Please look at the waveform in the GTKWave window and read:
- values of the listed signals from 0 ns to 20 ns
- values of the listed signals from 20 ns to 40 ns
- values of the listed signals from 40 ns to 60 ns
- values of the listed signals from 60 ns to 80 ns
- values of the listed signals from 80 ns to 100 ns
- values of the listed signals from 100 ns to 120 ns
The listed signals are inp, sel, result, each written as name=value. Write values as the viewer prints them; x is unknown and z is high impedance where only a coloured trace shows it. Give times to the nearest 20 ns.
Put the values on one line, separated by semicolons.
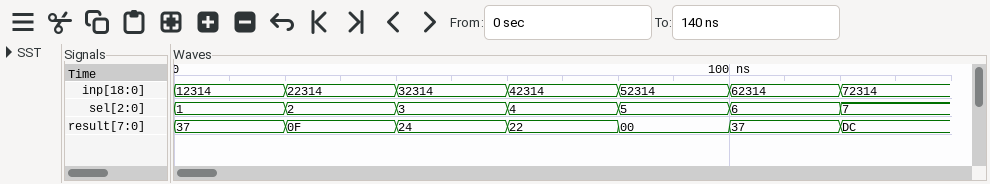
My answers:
inp=12314, sel=1, result=37; inp=22314, sel=2, result=0F; inp=32314, sel=3, result=24; inp=42314, sel=4, result=22; inp=52314, sel=5, result=00; inp=62314, sel=6, result=37
